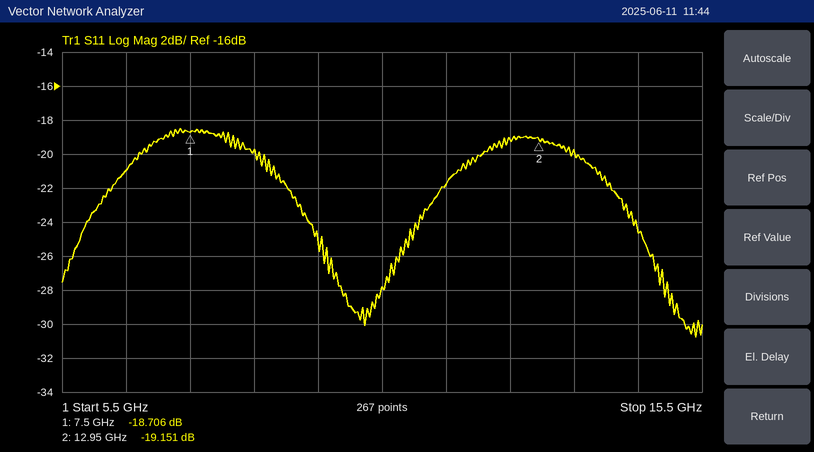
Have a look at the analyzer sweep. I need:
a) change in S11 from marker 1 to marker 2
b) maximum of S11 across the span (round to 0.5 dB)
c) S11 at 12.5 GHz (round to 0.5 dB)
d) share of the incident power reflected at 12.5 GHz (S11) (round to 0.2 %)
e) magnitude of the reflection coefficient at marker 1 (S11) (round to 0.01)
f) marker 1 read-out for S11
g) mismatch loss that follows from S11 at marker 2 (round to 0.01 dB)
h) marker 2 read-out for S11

-0.445 dB
-18.5 dB
-19.0 dB
1.2 %
0.12
-18.706 dB
0.05 dB
-19.151 dB
